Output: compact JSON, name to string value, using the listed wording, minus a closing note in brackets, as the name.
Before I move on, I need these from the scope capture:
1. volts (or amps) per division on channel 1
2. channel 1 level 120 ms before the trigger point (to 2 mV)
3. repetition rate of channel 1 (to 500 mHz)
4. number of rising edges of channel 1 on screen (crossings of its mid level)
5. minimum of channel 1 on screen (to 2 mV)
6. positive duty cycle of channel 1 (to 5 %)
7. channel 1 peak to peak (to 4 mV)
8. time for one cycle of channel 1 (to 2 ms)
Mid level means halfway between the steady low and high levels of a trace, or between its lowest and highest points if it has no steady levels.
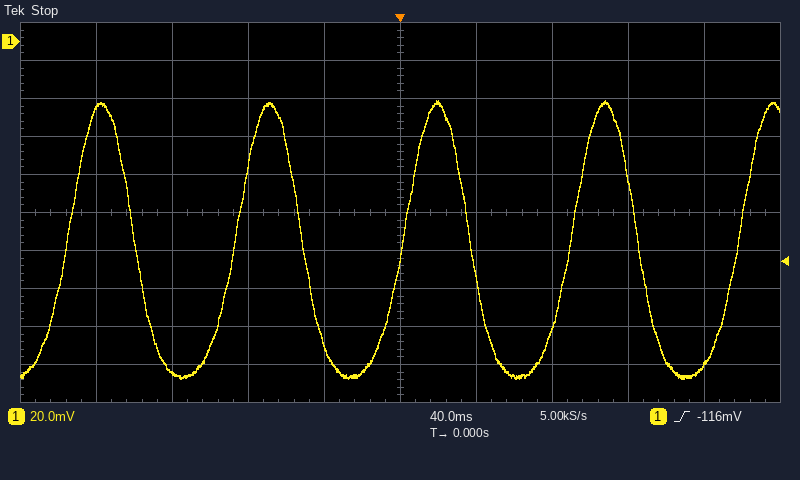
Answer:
{"volts (or amps) per division on channel 1": "20 mV", "channel 1 level 120 ms before the trigger point": "-174 mV", "repetition rate of channel 1": "11.5 Hz", "number of rising edges of channel 1 on screen": "5", "minimum of channel 1 on screen": "-178 mV", "positive duty cycle of channel 1": "40 %", "channel 1 peak to peak": "148 mV", "time for one cycle of channel 1": "88 ms"}
